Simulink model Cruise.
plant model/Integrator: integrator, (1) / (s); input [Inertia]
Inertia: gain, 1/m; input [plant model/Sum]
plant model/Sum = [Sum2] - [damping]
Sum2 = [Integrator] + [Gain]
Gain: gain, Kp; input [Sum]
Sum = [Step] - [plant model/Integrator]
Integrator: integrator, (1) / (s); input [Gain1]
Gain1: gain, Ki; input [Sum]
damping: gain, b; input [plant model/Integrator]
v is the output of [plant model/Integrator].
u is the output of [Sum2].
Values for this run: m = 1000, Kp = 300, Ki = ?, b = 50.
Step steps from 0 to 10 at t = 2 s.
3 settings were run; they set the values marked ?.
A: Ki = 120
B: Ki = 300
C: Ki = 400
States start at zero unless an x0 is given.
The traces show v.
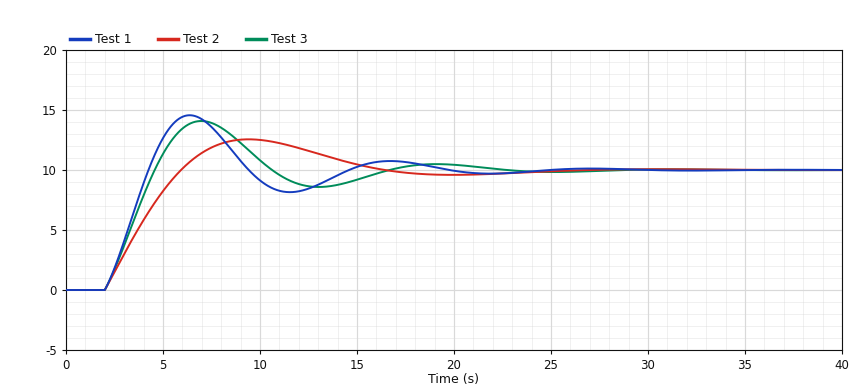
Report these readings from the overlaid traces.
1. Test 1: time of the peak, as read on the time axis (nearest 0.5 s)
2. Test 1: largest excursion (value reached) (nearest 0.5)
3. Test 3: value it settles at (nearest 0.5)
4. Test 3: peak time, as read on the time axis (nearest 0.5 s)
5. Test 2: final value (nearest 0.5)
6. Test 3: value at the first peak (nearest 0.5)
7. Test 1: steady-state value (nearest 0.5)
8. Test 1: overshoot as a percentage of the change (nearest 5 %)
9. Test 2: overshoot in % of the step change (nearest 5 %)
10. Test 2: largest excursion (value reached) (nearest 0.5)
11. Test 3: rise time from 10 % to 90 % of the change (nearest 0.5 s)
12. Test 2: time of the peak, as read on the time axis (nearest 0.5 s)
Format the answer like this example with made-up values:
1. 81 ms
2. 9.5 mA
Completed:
1. 6.5 s
2. 14.5
3. 10.0
4. 7.0 s
5. 10.0
6. 14.0
7. 10.0
8. 45 %
9. 25 %
10. 12.5
11. 2.0 s
12. 9.5 s
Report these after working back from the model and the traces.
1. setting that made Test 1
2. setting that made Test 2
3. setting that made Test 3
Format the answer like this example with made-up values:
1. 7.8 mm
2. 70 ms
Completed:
1. C
2. A
3. B
